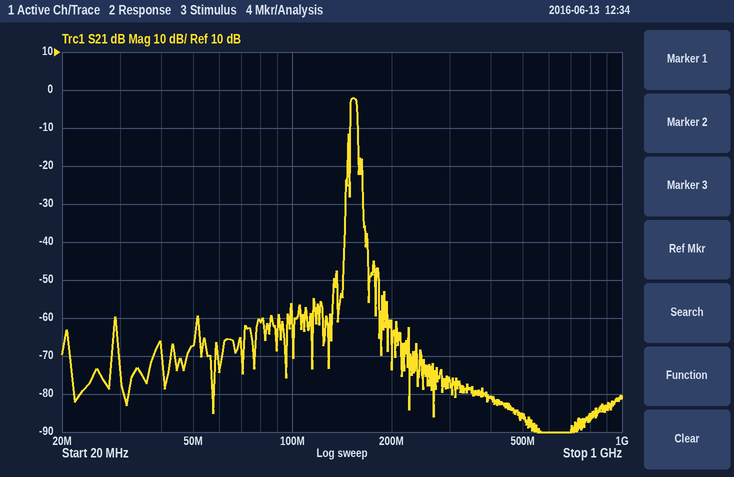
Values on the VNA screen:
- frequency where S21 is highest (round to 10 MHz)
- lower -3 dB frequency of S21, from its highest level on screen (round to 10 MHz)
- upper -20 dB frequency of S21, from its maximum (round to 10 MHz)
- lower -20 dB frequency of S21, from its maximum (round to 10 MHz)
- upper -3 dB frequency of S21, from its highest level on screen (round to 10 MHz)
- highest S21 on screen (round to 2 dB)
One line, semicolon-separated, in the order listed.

150 MHz; 150 MHz; 160 MHz; 150 MHz; 160 MHz; -2 dB
